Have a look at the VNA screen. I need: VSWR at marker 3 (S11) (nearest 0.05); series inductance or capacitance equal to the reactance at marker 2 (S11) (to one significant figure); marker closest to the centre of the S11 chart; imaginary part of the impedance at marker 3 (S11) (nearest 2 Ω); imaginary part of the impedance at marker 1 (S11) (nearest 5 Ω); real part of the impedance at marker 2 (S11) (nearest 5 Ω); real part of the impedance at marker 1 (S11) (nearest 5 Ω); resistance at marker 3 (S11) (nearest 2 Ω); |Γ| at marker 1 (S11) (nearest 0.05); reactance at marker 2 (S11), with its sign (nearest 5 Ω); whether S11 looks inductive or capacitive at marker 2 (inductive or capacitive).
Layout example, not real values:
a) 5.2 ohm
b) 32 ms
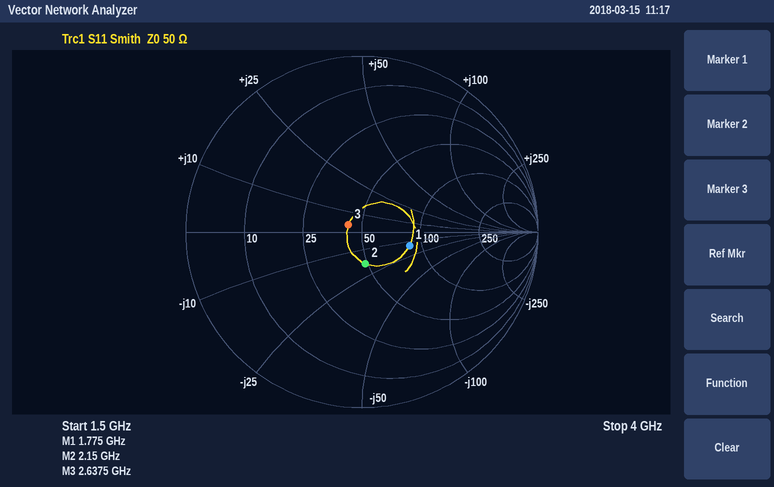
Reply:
a) 1.20
b) 4 pF
c) marker 3
d) +4 Ω
e) -15 Ω
f) 50 Ω
g) 85 Ω
h) 42 Ω
i) 0.30
j) -20 Ω
k) capacitive
